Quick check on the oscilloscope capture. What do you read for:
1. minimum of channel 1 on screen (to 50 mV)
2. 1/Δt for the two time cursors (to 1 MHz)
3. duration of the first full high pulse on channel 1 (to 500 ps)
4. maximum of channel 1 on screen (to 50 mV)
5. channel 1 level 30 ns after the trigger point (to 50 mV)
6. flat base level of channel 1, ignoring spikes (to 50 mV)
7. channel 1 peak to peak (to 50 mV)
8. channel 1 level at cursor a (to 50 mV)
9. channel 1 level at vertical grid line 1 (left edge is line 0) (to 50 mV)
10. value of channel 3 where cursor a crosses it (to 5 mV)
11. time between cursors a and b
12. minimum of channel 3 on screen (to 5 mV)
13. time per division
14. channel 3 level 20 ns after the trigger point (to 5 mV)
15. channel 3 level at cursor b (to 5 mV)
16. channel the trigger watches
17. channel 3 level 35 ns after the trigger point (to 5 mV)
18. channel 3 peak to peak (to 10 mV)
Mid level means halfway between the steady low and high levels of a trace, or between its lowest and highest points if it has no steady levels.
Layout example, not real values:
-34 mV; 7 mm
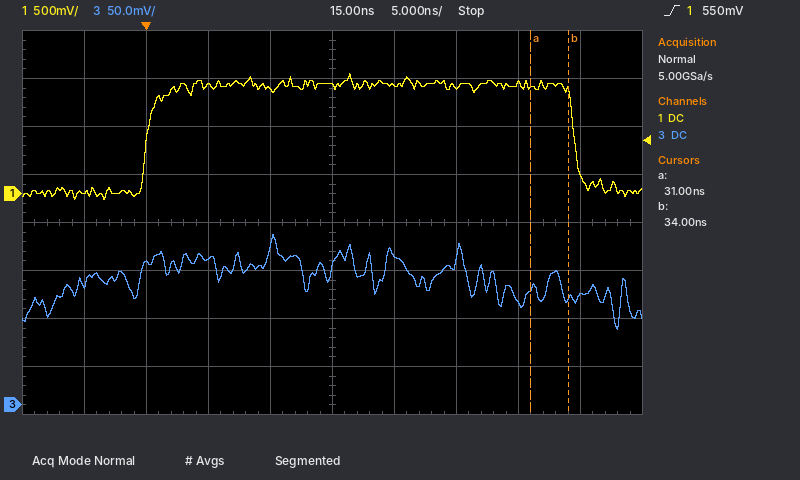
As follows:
-50 mV; 333 MHz; 34.5 ns; 1.25 V; 1.15 V; 0 mV; 1.30 V; 1.10 V; 0 mV; 120 mV; 3.0 ns; 80 mV; 5 ns; 155 mV; 110 mV; channel 1; 115 mV; 100 mV
